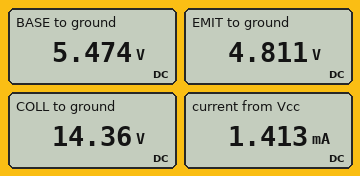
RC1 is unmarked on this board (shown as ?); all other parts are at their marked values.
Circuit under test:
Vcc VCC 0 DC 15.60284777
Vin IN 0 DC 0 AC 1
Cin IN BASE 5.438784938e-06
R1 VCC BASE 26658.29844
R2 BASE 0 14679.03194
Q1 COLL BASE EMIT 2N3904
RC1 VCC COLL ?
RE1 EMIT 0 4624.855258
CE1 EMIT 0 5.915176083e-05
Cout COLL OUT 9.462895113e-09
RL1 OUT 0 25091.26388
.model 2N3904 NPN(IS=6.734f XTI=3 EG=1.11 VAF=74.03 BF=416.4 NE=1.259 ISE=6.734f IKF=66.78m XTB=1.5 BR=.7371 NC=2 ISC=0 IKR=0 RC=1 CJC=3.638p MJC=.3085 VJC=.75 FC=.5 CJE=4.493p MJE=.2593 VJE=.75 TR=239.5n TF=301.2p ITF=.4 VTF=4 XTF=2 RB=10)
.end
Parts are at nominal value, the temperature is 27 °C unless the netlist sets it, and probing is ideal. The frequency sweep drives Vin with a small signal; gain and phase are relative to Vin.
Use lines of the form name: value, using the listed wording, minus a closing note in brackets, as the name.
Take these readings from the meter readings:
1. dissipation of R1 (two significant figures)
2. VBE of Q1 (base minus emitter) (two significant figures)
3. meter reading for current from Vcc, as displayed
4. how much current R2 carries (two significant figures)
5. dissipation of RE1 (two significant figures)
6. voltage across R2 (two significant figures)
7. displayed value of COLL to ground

dissipation of R1: 3.8 mW
VBE of Q1 (base minus emitter): 660 mV
meter reading for current from Vcc, as displayed: 1.413 mA
how much current R2 carries: 370 µA
dissipation of RE1: 5.0 mW
voltage across R2: 5.5 V
displayed value of COLL to ground: 14.36 V
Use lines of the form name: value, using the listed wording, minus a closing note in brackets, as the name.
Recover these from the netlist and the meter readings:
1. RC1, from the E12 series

RC1, from the E12 series: 1.2 kΩ
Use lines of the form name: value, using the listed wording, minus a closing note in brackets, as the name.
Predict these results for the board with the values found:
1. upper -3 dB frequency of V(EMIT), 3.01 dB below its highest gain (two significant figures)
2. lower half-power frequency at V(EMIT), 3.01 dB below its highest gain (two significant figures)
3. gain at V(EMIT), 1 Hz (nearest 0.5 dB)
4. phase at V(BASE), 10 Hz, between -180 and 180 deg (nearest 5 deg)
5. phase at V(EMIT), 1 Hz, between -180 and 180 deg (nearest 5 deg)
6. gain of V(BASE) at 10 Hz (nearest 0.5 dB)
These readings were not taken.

upper -3 dB frequency of V(EMIT), 3.01 dB below its highest gain: 120 Hz
lower half-power frequency at V(EMIT), 3.01 dB below its highest gain: 2.8 Hz
gain at V(EMIT), 1 Hz: -10.5 dB
phase at V(BASE), 10 Hz, between -180 and 180 deg: 15 deg
phase at V(EMIT), 1 Hz, between -180 and 180 deg: 70 deg
gain of V(BASE) at 10 Hz: -1.0 dB
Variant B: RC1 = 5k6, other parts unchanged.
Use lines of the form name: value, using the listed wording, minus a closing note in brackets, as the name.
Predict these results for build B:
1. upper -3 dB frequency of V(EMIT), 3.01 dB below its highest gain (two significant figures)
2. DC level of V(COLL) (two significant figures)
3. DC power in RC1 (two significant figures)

upper -3 dB frequency of V(EMIT), 3.01 dB below its highest gain: 110 Hz
DC level of V(COLL): 9.8 V
DC power in RC1: 6.0 mW
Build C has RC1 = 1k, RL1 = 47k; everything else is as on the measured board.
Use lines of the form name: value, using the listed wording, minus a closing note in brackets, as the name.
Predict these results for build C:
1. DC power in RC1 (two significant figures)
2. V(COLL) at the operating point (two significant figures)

DC power in RC1: 1.1 mW
V(COLL) at the operating point: 15 V
